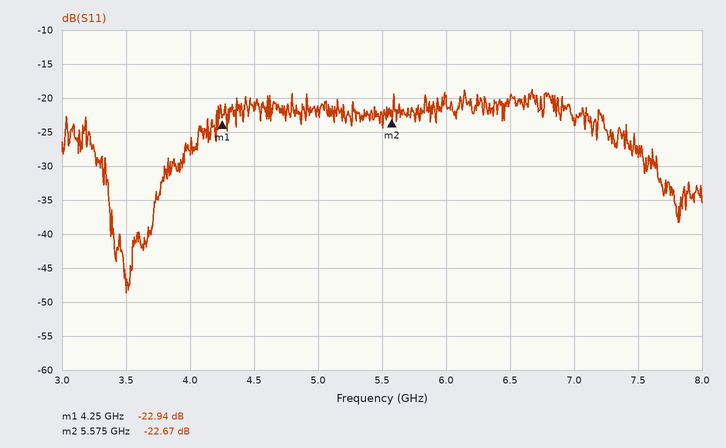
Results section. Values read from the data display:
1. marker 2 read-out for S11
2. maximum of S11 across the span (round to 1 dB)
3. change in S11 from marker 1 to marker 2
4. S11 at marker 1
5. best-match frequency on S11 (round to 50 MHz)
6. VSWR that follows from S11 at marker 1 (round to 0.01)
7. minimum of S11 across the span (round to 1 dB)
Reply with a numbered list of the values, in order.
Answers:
1. -22.67 dB
2. -19 dB
3. 0.27 dB
4. -22.94 dB
5. 3.50 GHz
6. 1.15
7. -49 dB
